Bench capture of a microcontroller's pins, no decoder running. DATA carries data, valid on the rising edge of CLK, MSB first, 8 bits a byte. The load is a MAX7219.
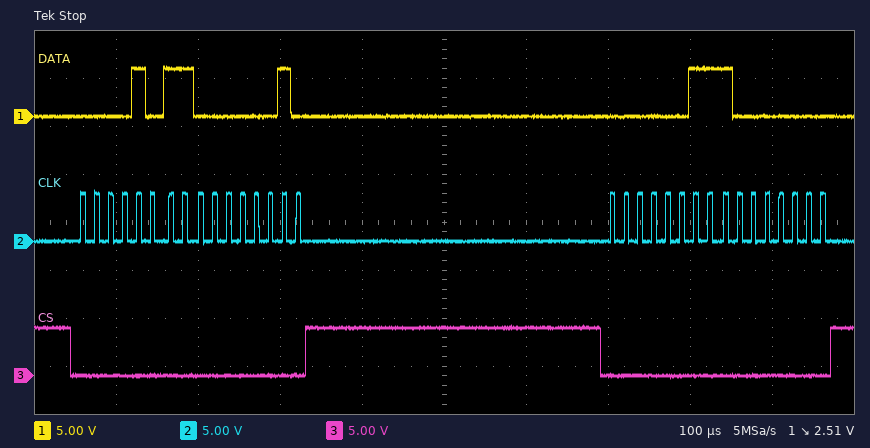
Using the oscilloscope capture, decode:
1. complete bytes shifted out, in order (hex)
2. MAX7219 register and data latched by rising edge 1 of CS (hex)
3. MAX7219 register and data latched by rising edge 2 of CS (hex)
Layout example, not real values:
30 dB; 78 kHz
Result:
0x0B 0x02 0x03 0x80; register 0xB, data 0x02; register 0x3, data 0x80
